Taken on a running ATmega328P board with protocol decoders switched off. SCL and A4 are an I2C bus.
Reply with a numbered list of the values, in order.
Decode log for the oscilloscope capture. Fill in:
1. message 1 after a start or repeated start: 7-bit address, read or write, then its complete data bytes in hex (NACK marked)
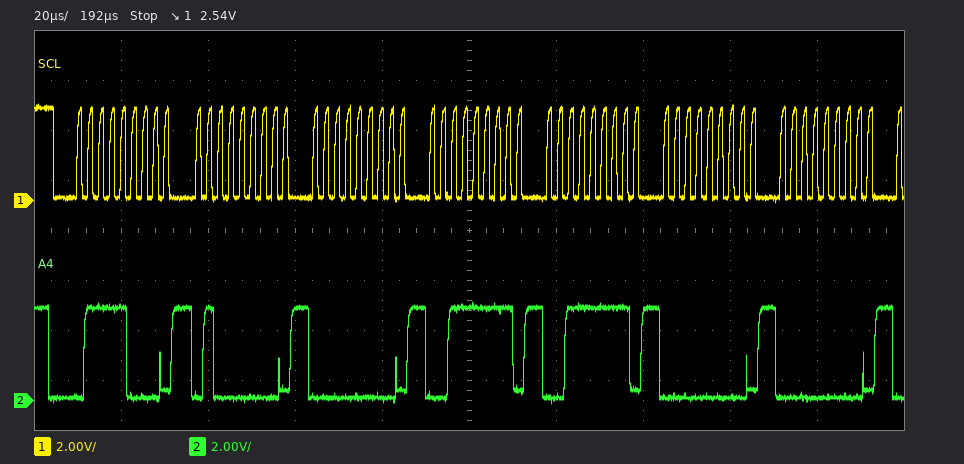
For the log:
1. 0x3C write: 40 00 3F 3F 00 00
